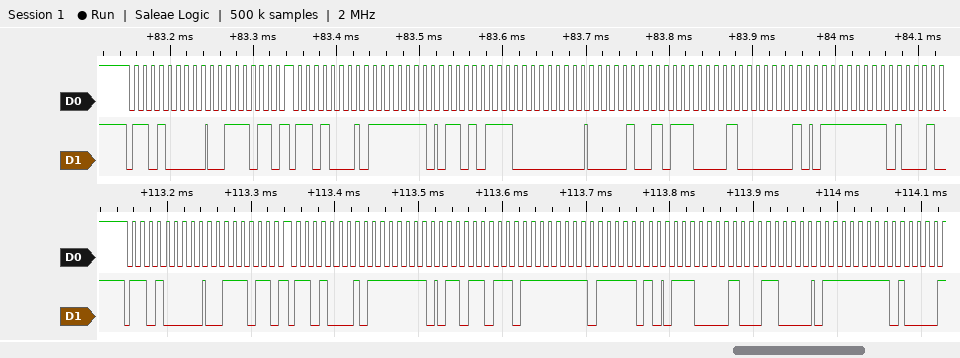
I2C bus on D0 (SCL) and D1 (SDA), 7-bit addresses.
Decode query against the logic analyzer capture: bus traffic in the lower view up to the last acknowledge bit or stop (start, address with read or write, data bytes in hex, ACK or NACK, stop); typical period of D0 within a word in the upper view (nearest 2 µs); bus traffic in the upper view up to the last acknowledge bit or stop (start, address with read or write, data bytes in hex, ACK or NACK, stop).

start, address 68 write ACK, 3B ACK, repeated start, address 68 read ACK, FE ACK, DB ACK, FF ACK, FA ACK, E1 ACK, 30 ACK, FF ACK
10 µs
start, address 68 write ACK, 3B ACK, repeated start, address 68 read ACK, FE ACK, D7 ACK, 00 ACK, 09 ACK, E1 ACK, 02 ACK, FF ACK
